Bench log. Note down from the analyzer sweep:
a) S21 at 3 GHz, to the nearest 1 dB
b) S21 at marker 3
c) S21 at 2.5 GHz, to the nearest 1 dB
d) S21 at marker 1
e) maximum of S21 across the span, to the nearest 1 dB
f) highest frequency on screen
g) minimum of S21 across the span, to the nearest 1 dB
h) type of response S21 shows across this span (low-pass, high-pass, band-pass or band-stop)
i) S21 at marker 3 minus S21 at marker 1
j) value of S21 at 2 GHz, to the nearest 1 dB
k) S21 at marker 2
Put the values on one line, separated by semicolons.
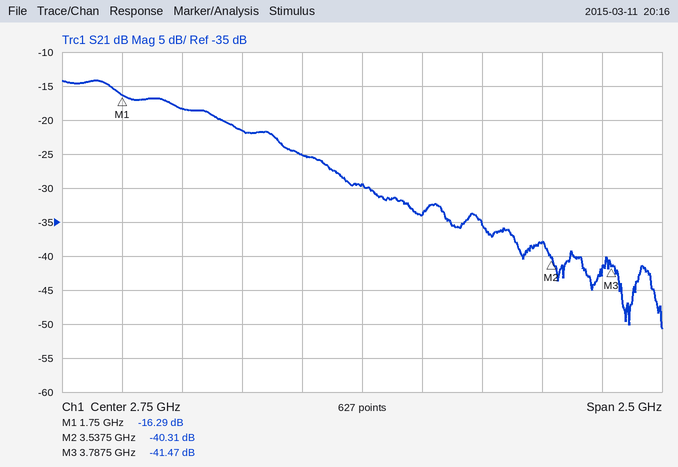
-34 dB; -41.47 dB; -25 dB; -16.29 dB; -14 dB; 4 GHz; -51 dB; low-pass; -25.18 dB; -18 dB; -40.31 dB
